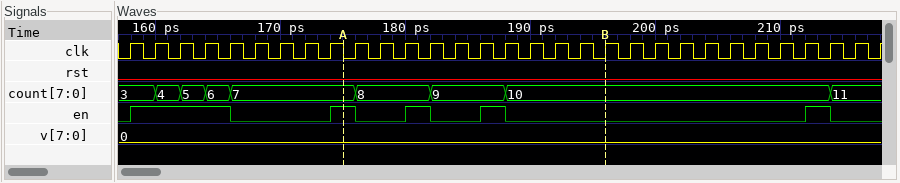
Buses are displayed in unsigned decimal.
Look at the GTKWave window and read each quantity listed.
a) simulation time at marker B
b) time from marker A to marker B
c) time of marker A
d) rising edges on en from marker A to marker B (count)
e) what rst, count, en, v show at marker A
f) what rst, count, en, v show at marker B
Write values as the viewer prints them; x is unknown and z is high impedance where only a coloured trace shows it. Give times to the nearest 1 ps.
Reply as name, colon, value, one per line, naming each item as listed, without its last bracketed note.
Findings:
simulation time at marker B: 196 ps
time from marker A to marker B: 21 ps
time of marker A: 175 ps
rising edges on en from marker A to marker B: 2
what rst, count, en, v show at marker A: rst=0, count=7, en=1, v=0
what rst, count, en, v show at marker B: rst=0, count=10, en=0, v=0
